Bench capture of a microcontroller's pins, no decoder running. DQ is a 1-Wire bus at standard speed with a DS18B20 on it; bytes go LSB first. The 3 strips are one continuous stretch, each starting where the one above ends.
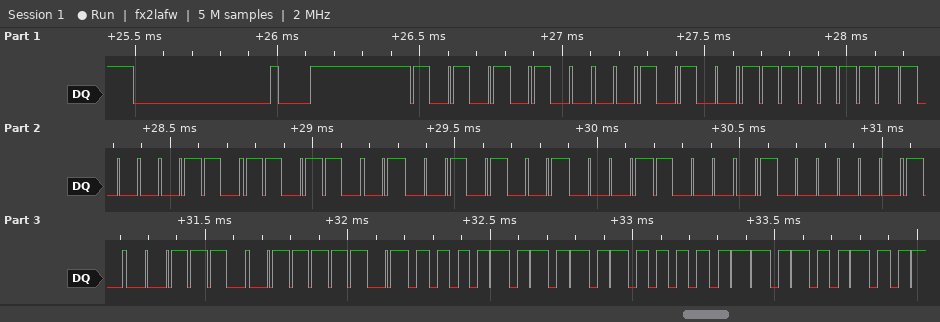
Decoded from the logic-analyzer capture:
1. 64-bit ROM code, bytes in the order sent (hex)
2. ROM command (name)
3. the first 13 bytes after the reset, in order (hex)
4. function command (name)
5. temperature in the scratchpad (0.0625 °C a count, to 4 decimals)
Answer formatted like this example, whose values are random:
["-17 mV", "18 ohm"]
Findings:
["28 FF 61 9B 94 18 02 71", "Match ROM", "55 28 FF 61 9B 94 18 02 71 BE 50 05 4B", "Read Scratchpad", "85.0000 °C"]
